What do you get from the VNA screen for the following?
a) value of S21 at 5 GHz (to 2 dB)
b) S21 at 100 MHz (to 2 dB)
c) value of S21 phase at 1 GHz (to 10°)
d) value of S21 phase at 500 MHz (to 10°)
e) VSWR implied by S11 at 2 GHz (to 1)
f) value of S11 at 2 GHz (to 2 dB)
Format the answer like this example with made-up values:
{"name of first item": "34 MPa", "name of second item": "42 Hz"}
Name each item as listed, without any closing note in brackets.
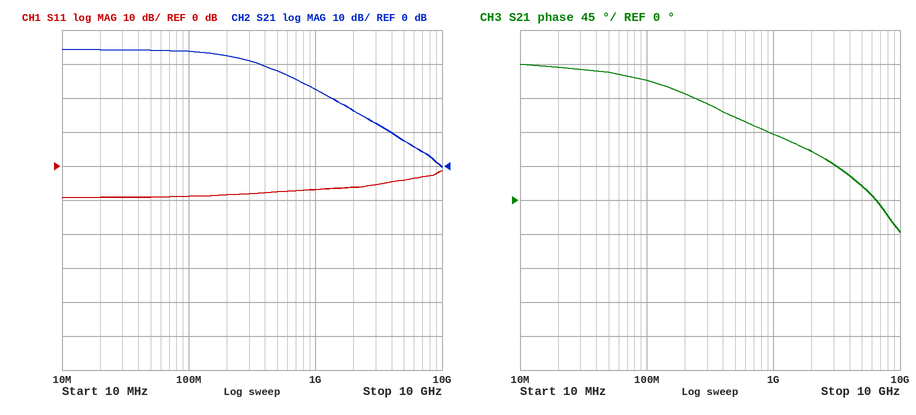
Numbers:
{"value of S21 at 5 GHz": "8 dB", "S21 at 100 MHz": "34 dB", "value of S21 phase at 1 GHz": "90°", "value of S21 phase at 500 MHz": "110°", "VSWR implied by S11 at 2 GHz": "3", "value of S11 at 2 GHz": "-6 dB"}
